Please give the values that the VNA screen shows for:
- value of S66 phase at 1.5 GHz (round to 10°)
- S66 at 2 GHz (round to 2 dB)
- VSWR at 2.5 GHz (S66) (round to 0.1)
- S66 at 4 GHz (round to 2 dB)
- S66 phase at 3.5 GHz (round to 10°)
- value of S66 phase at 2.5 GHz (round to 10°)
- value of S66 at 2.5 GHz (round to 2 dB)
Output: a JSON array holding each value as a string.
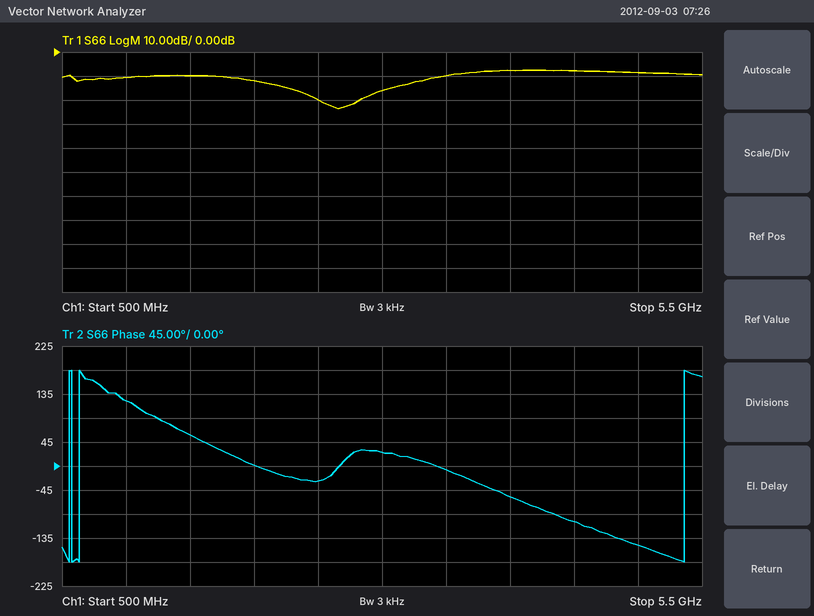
["60°", "-12 dB", "1.2", "-8 dB", "-10°", "-30°", "-20 dB"]
